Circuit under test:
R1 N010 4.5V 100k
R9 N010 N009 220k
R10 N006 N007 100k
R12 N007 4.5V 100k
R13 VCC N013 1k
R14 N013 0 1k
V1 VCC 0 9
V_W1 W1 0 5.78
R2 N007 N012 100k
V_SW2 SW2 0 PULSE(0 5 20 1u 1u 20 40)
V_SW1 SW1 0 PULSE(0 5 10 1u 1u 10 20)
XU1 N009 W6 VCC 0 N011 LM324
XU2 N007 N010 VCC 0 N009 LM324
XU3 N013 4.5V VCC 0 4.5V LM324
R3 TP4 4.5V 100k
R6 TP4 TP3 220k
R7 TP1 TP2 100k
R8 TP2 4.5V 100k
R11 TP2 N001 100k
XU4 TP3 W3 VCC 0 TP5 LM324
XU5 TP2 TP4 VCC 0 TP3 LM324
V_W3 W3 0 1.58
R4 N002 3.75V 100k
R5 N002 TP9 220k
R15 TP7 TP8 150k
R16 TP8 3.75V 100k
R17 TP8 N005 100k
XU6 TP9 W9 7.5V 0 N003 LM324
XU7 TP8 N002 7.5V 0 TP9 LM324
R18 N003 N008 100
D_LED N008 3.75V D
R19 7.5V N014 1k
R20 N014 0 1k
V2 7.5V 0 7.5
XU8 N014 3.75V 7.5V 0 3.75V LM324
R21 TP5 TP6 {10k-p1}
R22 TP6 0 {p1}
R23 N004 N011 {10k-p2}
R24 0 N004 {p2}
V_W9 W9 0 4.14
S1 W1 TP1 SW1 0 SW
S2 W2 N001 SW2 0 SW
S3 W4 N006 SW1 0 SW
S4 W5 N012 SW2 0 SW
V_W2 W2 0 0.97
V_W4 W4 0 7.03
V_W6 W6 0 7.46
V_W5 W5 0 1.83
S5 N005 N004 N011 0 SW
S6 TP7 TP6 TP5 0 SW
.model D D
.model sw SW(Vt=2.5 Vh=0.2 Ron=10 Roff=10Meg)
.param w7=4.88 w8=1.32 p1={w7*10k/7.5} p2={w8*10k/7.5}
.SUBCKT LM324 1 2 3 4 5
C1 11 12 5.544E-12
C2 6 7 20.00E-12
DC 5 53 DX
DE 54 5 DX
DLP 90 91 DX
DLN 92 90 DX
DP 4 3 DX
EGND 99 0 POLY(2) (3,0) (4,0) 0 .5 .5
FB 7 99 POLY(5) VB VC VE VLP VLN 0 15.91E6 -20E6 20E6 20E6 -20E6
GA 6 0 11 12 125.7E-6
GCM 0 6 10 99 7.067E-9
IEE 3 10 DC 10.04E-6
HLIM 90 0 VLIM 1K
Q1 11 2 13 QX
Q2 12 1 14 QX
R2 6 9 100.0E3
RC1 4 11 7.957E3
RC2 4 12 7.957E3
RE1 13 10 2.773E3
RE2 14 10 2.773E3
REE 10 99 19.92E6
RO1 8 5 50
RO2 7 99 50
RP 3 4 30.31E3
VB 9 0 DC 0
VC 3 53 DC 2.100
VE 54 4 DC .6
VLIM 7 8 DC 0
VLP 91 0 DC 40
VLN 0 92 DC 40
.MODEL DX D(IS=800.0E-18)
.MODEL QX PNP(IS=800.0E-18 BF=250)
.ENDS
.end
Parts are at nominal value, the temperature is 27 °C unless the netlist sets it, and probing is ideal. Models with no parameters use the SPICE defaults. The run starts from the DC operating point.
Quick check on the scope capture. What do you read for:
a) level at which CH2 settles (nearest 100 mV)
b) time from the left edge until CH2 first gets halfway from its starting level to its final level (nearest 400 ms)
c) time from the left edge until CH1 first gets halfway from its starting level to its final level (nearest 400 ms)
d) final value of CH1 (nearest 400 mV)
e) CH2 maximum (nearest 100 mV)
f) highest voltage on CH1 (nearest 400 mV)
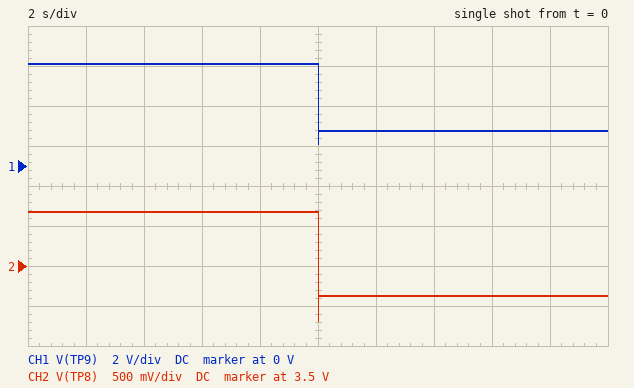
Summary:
3.1 V
10.0 s
10.0 s
1.6 V
4.2 V
5.2 V
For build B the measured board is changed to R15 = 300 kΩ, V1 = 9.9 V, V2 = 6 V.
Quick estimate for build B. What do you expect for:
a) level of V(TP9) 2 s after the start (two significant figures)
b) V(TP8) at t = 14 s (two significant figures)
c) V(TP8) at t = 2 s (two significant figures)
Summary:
4.5 V
2.7 V
3.6 V
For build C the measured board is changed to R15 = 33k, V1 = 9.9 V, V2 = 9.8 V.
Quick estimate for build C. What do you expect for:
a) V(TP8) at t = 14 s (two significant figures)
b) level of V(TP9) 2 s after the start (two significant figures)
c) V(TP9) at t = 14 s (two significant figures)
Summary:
4.5 V
6.2 V
3.7 V
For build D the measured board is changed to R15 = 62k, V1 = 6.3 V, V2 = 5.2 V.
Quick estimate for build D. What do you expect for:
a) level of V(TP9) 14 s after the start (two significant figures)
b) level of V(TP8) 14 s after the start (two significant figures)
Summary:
3.6 V
2.9 V
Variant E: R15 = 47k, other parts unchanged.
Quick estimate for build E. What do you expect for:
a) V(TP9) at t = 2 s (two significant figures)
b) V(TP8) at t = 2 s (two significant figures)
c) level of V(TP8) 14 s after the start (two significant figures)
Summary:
6.0 V
4.5 V
3.7 V
